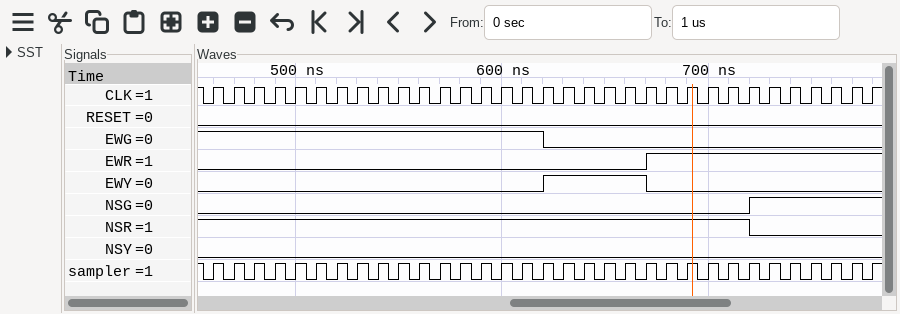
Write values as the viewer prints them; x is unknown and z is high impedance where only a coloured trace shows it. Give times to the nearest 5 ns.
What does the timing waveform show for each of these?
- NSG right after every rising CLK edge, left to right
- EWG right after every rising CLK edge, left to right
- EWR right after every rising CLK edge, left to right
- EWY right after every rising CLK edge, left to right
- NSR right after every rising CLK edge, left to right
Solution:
0 0 0 0 0 0 0 0 0 0 0 0 0 0 0 0 0 0 0 0 0 0 0 0 0 0 1 1 1 1 1 1 1
1 1 1 1 1 1 1 1 1 1 1 1 1 1 1 1 0 0 0 0 0 0 0 0 0 0 0 0 0 0 0 0 0
0 0 0 0 0 0 0 0 0 0 0 0 0 0 0 0 0 0 0 0 0 1 1 1 1 1 1 1 1 1 1 1 1
0 0 0 0 0 0 0 0 0 0 0 0 0 0 0 0 1 1 1 1 1 0 0 0 0 0 0 0 0 0 0 0 0
1 1 1 1 1 1 1 1 1 1 1 1 1 1 1 1 1 1 1 1 1 1 1 1 1 1 0 0 0 0 0 0 0
